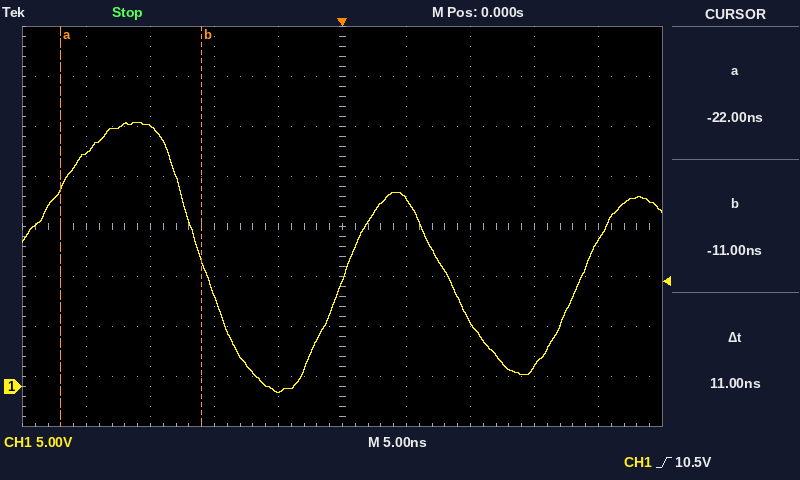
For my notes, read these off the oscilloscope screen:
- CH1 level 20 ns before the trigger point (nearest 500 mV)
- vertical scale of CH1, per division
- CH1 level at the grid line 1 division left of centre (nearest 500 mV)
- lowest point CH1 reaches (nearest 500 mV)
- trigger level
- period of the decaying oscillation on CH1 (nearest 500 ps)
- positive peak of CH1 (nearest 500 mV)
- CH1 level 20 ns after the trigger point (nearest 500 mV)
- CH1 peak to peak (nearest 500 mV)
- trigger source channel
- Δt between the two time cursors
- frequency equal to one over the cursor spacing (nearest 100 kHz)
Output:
23.5 V
5 V
-500 mV
-500 mV
10.5 V
19.5 ns
26.5 V
14.5 V
27.0 V
CH1
11 ns
90.9 MHz
